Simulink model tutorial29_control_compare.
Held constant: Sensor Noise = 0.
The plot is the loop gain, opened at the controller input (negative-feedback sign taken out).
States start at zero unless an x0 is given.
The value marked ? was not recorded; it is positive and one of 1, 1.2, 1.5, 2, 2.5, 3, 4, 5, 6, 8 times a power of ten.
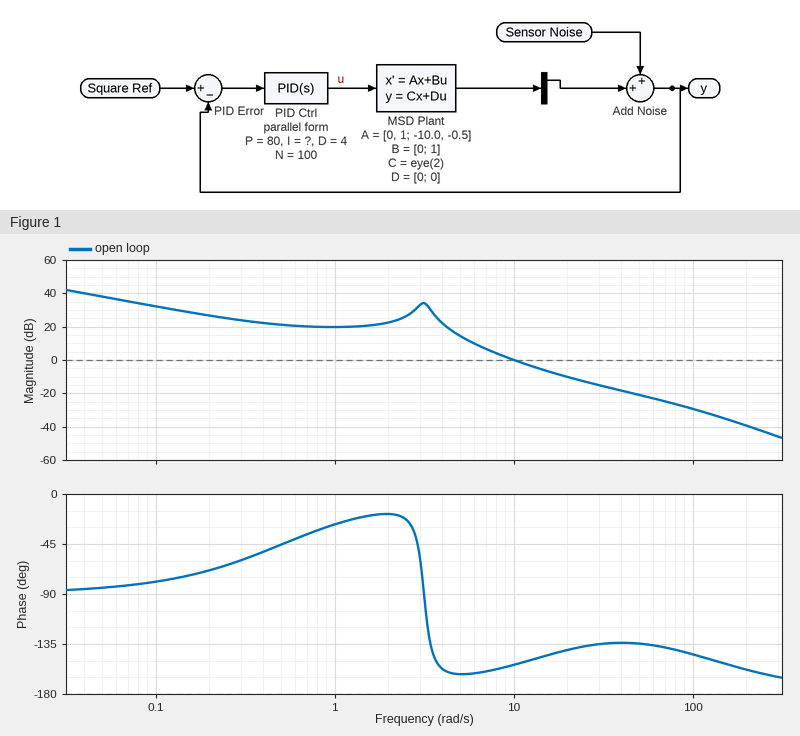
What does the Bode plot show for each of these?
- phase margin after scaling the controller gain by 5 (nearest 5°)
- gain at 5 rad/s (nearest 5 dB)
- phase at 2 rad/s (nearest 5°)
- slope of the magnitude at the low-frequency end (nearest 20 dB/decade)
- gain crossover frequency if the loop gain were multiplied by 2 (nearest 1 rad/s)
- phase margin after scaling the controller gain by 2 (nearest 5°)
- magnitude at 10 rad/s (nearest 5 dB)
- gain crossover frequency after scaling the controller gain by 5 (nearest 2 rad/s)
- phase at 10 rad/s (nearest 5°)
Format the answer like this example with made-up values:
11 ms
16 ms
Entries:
45°
15 dB
-20°
-20 dB/decade
15 rad/s
35°
0 dB
28 rad/s
-155°
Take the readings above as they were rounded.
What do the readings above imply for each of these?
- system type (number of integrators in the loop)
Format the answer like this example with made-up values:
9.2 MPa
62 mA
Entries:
1
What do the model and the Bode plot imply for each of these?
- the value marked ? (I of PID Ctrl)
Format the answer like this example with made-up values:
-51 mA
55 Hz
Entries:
40
